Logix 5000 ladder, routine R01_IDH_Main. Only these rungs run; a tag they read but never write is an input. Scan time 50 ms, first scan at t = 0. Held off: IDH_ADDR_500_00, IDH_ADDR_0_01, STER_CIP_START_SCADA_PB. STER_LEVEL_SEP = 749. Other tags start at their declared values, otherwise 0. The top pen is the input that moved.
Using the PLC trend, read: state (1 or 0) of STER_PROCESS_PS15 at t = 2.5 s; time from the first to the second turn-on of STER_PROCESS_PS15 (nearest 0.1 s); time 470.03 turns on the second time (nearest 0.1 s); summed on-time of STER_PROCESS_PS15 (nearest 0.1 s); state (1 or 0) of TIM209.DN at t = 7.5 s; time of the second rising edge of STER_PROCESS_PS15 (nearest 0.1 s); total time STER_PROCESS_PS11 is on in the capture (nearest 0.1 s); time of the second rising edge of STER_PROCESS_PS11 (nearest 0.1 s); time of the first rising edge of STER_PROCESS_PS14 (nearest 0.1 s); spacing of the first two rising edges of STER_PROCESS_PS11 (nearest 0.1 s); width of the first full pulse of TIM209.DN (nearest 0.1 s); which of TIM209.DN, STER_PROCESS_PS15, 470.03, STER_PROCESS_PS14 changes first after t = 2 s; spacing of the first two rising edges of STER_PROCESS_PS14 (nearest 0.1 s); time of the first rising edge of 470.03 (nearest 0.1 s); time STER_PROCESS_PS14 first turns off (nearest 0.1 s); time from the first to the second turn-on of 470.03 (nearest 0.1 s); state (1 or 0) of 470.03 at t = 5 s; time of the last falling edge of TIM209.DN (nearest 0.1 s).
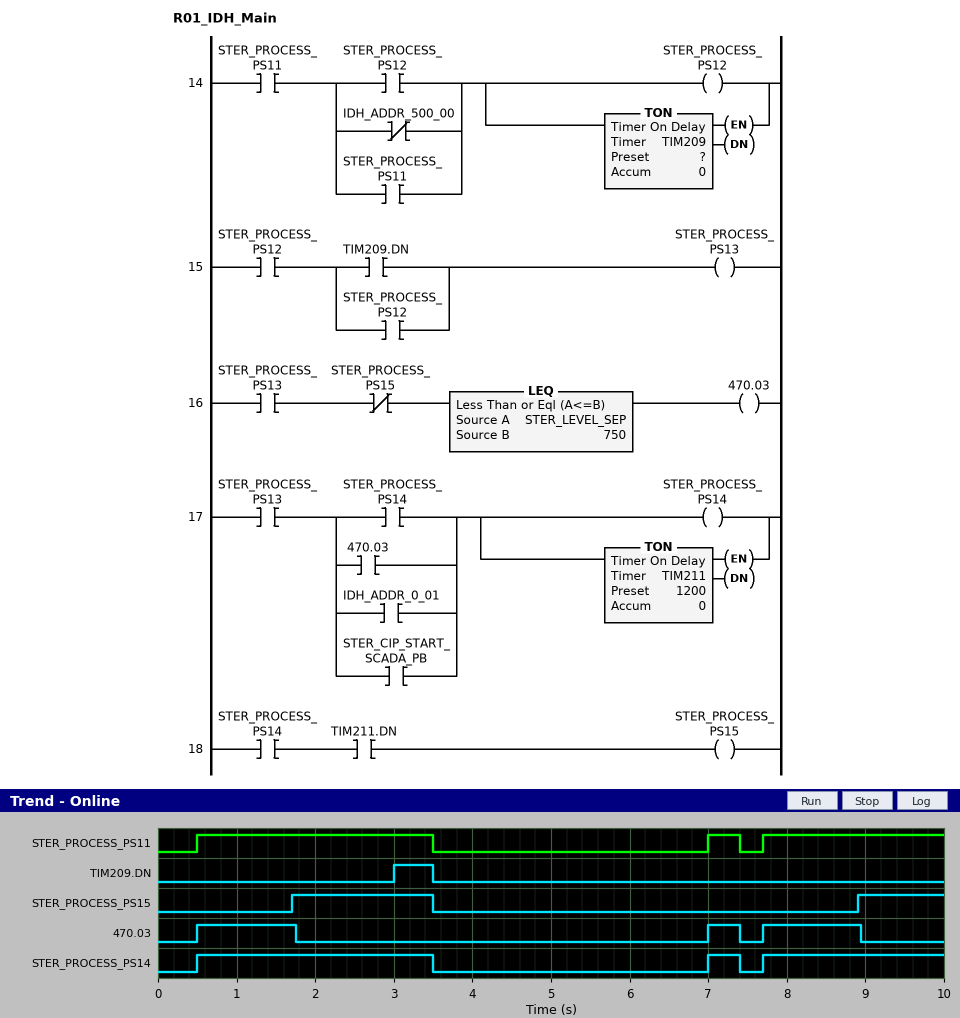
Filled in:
1
7.2 s
7.0 s
2.9 s
0
8.9 s
5.7 s
7.0 s
0.5 s
6.5 s
0.5 s
TIM209.DN
6.5 s
0.5 s
3.5 s
6.5 s
0
3.5 s
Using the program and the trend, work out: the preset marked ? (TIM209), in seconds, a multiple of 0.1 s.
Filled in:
2.5 s
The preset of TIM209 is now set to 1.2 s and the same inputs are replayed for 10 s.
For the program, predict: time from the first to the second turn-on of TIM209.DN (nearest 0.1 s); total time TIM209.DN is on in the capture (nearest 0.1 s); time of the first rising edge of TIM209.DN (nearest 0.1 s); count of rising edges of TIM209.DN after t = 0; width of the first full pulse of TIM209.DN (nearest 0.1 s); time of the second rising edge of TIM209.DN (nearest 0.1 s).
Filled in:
7.2 s
2.9 s
1.7 s
2
1.8 s
8.9 s
